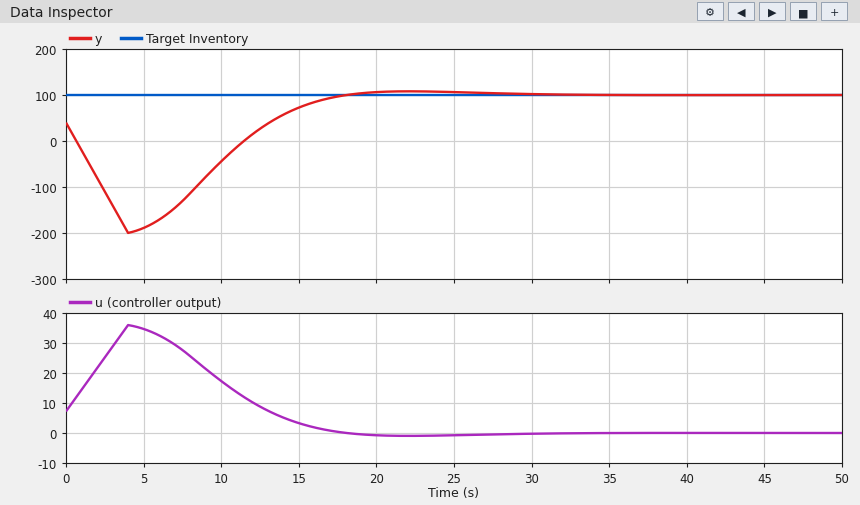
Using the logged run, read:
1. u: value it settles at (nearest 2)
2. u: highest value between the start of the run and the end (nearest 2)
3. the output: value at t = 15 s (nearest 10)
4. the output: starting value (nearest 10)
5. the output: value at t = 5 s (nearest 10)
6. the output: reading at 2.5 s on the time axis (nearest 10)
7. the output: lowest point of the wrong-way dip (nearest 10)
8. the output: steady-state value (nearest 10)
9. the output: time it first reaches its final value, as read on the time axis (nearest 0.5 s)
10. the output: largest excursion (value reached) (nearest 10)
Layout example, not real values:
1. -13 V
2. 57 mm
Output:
1. 0
2. 36
3. 70
4. 40
5. -190
6. -110
7. -200
8. 100
9. 18.0 s
10. 110
